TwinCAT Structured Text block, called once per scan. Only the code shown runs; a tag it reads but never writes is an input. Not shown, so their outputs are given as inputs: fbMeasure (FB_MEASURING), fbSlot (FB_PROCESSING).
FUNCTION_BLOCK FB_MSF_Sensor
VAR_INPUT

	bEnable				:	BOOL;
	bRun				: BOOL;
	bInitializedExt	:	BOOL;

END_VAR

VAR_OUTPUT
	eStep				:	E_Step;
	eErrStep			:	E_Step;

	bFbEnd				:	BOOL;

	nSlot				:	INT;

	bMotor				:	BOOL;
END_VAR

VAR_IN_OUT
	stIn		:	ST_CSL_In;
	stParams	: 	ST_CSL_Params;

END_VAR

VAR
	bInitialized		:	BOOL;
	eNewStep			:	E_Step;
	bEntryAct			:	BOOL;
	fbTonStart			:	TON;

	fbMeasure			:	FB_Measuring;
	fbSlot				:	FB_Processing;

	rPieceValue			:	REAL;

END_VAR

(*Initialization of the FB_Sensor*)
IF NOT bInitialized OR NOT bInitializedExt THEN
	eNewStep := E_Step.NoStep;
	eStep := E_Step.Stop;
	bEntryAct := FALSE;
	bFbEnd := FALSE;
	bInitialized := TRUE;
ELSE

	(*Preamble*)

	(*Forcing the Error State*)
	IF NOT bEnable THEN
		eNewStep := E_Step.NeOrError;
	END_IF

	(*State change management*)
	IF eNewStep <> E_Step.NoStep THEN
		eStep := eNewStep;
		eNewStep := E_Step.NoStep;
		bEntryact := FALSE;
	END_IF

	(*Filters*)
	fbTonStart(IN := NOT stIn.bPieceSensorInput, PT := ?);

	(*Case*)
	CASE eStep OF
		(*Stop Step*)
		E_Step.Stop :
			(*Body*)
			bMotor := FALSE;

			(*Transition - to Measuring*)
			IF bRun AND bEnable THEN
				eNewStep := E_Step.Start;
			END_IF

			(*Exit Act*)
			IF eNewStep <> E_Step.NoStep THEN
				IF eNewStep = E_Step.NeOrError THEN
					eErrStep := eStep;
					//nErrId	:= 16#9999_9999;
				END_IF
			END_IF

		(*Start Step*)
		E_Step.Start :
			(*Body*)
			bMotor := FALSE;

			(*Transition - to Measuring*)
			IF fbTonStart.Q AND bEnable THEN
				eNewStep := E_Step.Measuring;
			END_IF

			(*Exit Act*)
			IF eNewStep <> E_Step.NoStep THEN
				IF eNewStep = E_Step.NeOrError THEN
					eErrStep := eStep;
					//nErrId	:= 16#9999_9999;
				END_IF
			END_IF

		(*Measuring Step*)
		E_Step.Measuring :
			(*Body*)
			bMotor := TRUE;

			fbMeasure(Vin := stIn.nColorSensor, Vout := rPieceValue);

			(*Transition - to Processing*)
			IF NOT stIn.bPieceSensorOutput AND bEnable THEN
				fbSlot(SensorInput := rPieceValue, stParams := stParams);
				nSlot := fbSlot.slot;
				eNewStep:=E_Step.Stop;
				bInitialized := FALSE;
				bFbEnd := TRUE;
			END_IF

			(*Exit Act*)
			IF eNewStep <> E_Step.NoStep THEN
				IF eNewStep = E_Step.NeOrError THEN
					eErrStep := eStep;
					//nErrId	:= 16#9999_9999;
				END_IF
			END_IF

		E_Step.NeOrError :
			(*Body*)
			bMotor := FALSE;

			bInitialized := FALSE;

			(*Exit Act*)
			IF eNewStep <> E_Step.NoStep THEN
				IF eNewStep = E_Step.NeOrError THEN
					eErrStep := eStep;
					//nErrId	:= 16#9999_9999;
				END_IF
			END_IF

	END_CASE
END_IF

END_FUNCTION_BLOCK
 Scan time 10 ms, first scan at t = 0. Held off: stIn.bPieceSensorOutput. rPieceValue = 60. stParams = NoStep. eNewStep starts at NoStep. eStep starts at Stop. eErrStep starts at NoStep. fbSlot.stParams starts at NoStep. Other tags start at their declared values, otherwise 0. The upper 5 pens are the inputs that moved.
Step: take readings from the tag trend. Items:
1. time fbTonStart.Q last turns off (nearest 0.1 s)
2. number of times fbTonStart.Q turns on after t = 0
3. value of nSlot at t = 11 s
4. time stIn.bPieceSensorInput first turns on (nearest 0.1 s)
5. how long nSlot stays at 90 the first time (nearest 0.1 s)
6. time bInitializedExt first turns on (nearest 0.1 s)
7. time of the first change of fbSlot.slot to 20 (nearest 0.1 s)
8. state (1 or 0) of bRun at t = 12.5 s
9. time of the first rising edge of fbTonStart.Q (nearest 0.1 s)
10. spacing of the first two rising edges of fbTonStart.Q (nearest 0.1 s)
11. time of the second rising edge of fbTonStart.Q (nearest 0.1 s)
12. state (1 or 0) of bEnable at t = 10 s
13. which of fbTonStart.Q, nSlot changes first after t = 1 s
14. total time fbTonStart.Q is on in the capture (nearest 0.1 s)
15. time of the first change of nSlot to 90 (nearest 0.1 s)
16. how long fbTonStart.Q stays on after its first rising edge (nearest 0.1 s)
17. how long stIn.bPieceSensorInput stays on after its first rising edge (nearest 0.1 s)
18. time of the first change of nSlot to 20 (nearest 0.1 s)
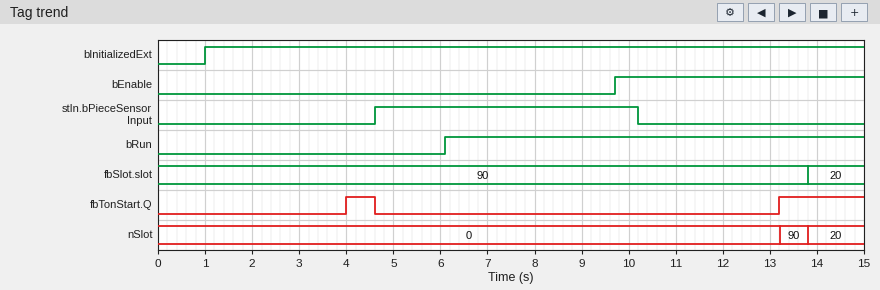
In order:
4.6 s
2
0
4.6 s
0.6 s
1.0 s
13.8 s
1
4.0 s
9.2 s
13.2 s
1
fbTonStart.Q
2.4 s
13.2 s
0.6 s
5.6 s
13.8 s
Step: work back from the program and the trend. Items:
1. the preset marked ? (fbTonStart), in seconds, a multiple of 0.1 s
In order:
3.0 s
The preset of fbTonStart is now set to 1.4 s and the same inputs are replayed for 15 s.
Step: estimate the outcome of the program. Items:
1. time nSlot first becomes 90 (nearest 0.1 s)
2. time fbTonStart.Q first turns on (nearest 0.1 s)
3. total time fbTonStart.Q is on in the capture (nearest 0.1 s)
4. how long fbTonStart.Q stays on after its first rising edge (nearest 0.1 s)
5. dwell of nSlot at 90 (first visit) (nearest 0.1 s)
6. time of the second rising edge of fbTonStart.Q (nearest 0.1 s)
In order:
11.6 s
2.4 s
5.6 s
2.2 s
2.2 s
11.6 s
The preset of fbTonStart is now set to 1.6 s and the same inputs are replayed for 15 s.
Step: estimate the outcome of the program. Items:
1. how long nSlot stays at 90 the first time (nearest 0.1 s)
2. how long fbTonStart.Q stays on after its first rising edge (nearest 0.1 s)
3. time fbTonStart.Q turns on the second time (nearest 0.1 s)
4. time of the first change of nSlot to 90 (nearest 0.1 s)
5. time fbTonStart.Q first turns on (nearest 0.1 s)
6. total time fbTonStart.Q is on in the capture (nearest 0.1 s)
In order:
2.0 s
2.0 s
11.8 s
11.8 s
2.6 s
5.2 s
